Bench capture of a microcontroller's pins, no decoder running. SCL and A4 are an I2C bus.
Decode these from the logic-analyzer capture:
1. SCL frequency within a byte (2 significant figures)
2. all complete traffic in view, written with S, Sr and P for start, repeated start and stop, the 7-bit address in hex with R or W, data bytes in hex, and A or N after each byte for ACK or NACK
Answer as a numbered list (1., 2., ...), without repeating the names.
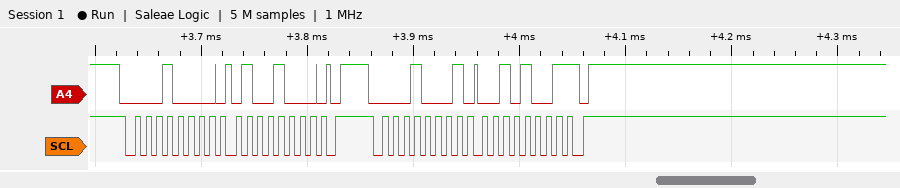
1. 100 kHz
2. S 08W A 48 A P S 08R A 29 N P
